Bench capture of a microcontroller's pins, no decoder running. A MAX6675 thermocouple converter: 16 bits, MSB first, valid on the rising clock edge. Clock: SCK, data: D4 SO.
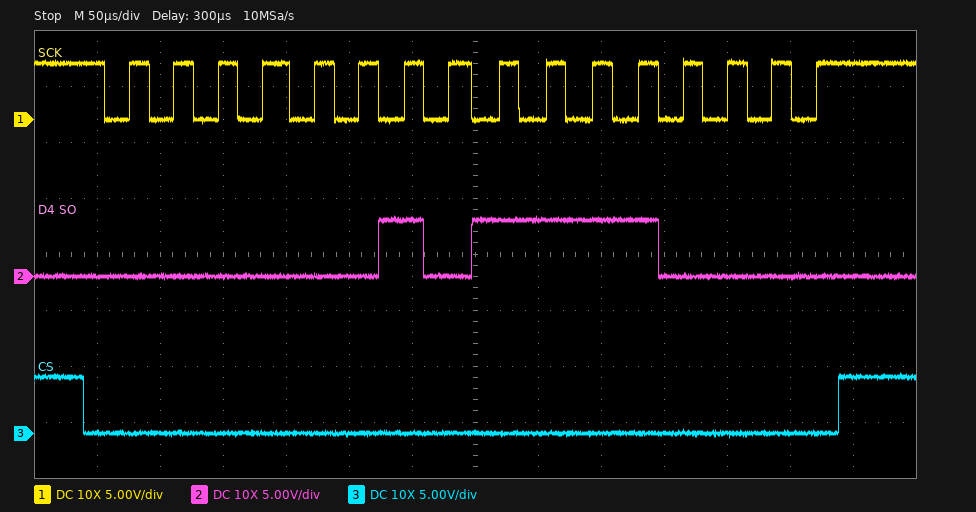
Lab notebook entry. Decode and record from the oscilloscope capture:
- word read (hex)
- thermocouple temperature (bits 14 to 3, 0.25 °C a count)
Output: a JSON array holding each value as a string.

["0x02F0", "23.50 °C"]
